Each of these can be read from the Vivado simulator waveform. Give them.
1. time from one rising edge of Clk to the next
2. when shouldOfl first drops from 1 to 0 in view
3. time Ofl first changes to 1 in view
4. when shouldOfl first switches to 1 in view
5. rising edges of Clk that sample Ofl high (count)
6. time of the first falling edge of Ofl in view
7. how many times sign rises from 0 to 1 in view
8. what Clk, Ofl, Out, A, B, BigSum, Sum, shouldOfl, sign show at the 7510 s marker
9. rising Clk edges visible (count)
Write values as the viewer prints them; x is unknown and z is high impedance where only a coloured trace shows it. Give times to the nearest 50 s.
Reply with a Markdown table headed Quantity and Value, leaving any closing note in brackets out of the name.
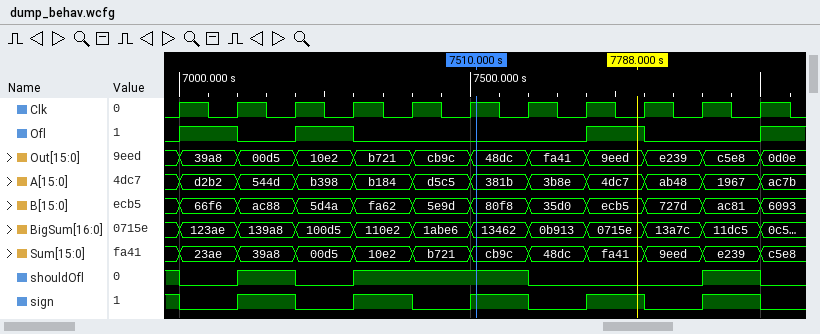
| Quantity | Value |
|---|---|
| time from one rising edge of Clk to the next | 100 s |
| when shouldOfl first drops from 1 to 0 in view | 7000 s |
| time Ofl first changes to 1 in view | 7000 s |
| when shouldOfl first switches to 1 in view | 7100 s |
| rising edges of Clk that sample Ofl high | 3 |
| time of the first falling edge of Ofl in view | 7100 s |
| how many times sign rises from 0 to 1 in view | 5 |
| what Clk, Ofl, Out, A, B, BigSum, Sum, shouldOfl, sign show at the 7510 s marker | Clk=1, Ofl=0, Out=48dc, A=381b, B=80f8, BigSum=13462, Sum=cb9c, shouldOfl=1, sign=1 |
| rising Clk edges visible | 11 |
